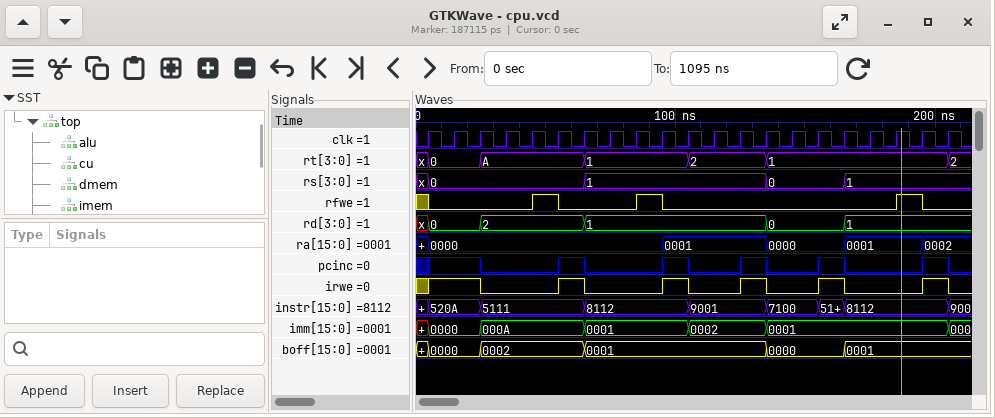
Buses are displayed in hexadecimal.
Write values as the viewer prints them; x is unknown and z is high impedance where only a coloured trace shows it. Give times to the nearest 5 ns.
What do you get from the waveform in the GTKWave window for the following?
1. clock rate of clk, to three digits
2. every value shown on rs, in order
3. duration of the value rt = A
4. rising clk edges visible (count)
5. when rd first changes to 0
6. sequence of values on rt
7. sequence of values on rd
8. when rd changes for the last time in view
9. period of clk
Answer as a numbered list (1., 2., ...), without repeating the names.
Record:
1. 100 MHz
2. x, 0, 1, 0, 1
3. 40 ns
4. 21
5. 5 ns
6. x, 0, A, 1, 2, 1, 2
7. x, 0, 2, 1, 0, 1
8. 165 ns
9. 10 ns
